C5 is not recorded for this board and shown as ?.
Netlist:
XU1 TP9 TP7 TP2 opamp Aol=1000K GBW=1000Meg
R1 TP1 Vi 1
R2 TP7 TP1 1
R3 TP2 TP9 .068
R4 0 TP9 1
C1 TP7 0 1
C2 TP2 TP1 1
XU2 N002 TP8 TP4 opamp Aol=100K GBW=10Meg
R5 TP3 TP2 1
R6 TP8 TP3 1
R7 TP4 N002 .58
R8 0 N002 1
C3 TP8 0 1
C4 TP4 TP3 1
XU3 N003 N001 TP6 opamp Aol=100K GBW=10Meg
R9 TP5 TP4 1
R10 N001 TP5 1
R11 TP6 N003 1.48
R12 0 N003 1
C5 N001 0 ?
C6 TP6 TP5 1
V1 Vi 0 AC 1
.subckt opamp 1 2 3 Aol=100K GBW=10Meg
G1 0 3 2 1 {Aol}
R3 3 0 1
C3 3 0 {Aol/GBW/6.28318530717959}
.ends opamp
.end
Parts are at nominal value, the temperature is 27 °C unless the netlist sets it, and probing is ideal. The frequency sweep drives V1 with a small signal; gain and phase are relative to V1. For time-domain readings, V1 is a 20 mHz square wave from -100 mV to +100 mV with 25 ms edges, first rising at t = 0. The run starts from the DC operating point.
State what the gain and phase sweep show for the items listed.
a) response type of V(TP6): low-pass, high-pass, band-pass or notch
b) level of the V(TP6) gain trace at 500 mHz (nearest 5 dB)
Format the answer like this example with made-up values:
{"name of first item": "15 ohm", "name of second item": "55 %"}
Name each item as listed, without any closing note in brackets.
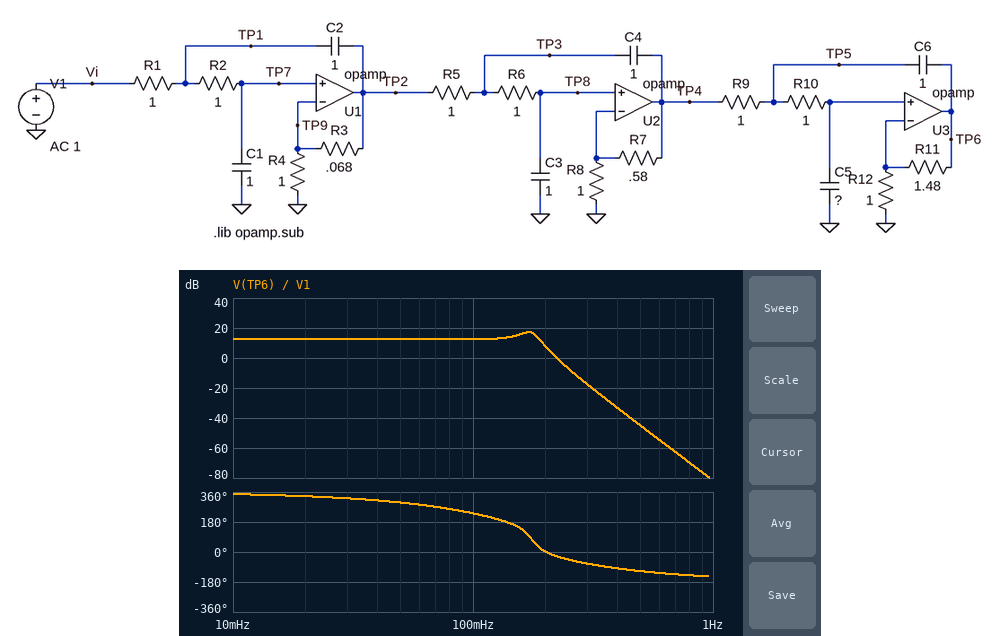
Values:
{"response type of V(TP6): low-pass, high-pass, band-pass or notch": "low-pass", "level of the V(TP6) gain trace at 500 mHz": "-45 dB"}
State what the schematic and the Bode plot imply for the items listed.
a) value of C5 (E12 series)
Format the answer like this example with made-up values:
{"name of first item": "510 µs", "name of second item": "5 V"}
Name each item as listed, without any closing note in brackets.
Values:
{"value of C5": "820 mF"}
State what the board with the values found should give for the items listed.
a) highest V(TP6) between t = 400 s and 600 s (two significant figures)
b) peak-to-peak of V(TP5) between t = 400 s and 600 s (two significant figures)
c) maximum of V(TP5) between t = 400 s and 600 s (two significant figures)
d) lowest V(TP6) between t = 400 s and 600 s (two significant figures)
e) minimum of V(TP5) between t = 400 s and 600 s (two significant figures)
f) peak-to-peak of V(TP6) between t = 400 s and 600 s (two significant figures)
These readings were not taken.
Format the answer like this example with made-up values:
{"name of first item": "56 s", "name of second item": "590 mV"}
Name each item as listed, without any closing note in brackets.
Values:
{"highest V(TP6) between t = 400 s and 600 s": "600 mV", "peak-to-peak of V(TP5) between t = 400 s and 600 s": "550 mV", "maximum of V(TP5) between t = 400 s and 600 s": "280 mV", "lowest V(TP6) between t = 400 s and 600 s": "-600 mV", "minimum of V(TP5) between t = 400 s and 600 s": "-280 mV", "peak-to-peak of V(TP6) between t = 400 s and 600 s": "1.2 V"}
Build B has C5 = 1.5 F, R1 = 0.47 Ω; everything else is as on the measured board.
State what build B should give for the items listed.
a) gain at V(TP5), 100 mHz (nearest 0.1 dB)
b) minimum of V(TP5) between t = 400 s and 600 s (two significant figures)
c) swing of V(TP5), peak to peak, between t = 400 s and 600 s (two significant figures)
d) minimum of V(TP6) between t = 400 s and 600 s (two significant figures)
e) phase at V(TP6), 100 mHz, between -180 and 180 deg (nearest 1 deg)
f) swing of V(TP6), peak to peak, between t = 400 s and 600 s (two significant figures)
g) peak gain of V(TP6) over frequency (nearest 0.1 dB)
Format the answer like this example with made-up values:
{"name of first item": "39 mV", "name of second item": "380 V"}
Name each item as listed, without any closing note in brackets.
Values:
{"gain at V(TP5), 100 mHz": "4.6 dB", "minimum of V(TP5) between t = 400 s and 600 s": "-220 mV", "swing of V(TP5), peak to peak, between t = 400 s and 600 s": "440 mV", "minimum of V(TP6) between t = 400 s and 600 s": "-470 mV", "phase at V(TP6), 100 mHz, between -180 and 180 deg": "-171 deg", "swing of V(TP6), peak to peak, between t = 400 s and 600 s": "940 mV", "peak gain of V(TP6) over frequency": "12.4 dB"}
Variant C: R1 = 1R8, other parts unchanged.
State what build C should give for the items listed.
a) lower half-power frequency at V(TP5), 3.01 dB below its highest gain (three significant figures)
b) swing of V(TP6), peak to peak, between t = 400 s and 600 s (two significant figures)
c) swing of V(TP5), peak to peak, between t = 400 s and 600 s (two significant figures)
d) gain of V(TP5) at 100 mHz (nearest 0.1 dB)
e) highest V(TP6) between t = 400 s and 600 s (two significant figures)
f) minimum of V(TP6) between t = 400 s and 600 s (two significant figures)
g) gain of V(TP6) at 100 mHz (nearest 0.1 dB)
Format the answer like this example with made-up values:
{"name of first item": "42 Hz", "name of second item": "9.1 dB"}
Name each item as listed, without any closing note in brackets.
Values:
{"lower half-power frequency at V(TP5), 3.01 dB below its highest gain": "146 mHz", "swing of V(TP6), peak to peak, between t = 400 s and 600 s": "970 mV", "swing of V(TP5), peak to peak, between t = 400 s and 600 s": "430 mV", "gain of V(TP5) at 100 mHz": "3.6 dB", "highest V(TP6) between t = 400 s and 600 s": "480 mV", "minimum of V(TP6) between t = 400 s and 600 s": "-480 mV", "gain of V(TP6) at 100 mHz": "10.4 dB"}
